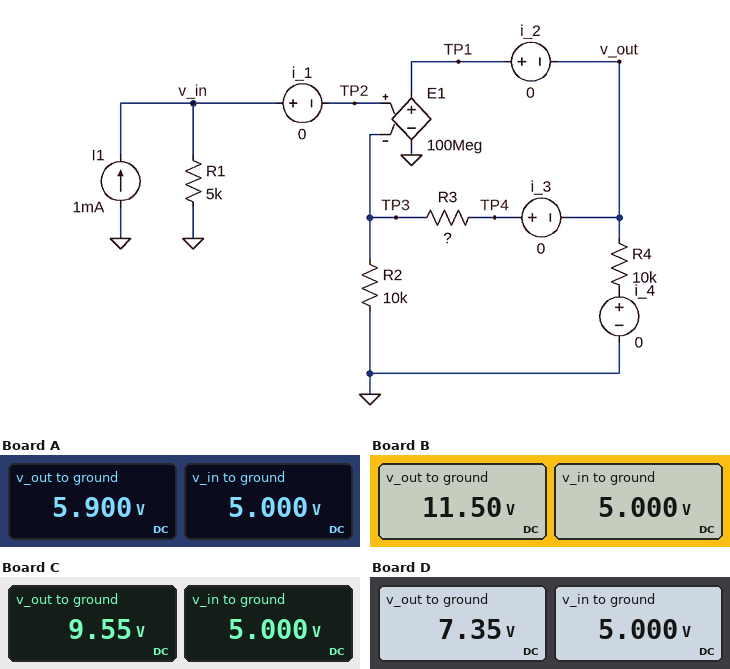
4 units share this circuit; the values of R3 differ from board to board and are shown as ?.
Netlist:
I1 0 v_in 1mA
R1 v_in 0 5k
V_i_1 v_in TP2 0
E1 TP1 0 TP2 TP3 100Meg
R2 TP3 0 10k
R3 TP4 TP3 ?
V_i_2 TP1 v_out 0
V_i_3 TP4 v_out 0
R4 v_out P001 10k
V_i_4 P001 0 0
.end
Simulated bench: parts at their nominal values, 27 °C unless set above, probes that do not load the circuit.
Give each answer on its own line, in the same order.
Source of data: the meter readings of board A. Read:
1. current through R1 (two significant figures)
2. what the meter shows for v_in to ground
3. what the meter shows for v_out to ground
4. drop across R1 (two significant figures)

1.0 mA
5.000 V
5.900 V
5.0 V
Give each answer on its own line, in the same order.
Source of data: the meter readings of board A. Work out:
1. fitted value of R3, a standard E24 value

1.8 kΩ
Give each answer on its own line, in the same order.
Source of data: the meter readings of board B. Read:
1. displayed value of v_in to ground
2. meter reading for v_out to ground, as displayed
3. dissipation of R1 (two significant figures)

5.000 V
11.50 V
5.0 mW
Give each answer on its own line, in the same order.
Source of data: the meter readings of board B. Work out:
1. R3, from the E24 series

13 kΩ
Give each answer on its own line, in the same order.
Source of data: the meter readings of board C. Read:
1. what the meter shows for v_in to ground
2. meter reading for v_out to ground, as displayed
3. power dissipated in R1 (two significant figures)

5.000 V
9.55 V
5.0 mW
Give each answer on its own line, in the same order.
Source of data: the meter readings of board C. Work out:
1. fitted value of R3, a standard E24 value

9.1 kΩ
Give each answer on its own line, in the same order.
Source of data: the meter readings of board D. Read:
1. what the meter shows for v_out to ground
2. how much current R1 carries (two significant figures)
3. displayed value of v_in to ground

7.35 V
1.0 mA
5.000 V
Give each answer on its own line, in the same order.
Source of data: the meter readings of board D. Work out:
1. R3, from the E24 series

4.7 kΩ
